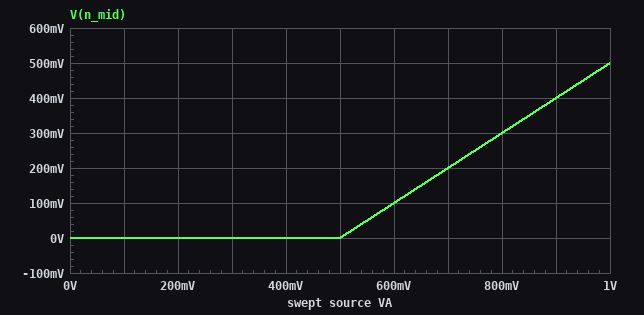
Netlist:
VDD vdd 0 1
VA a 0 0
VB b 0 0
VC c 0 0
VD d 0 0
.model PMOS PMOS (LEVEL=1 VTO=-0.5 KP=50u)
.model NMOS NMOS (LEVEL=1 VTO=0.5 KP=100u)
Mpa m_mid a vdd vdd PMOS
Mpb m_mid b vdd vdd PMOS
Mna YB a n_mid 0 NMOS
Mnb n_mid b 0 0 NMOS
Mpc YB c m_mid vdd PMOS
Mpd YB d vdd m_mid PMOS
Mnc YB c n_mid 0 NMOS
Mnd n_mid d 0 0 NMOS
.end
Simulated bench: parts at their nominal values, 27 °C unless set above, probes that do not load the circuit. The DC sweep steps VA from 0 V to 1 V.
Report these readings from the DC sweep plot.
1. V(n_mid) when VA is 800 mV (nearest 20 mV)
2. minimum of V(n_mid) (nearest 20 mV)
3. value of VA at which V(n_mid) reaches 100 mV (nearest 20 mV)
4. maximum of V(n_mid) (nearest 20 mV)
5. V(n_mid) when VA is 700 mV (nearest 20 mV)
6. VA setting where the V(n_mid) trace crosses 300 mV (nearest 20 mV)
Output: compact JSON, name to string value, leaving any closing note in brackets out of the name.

{"V(n_mid) when VA is 800 mV": "300 mV", "minimum of V(n_mid)": "0 V", "value of VA at which V(n_mid) reaches 100 mV": "600 mV", "maximum of V(n_mid)": "500 mV", "V(n_mid) when VA is 700 mV": "200 mV", "VA setting where the V(n_mid) trace crosses 300 mV": "800 mV"}
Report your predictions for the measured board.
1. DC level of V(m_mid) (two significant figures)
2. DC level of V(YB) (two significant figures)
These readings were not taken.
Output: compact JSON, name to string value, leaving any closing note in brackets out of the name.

{"DC level of V(m_mid)": "1.0 V", "DC level of V(YB)": "1.0 V"}
